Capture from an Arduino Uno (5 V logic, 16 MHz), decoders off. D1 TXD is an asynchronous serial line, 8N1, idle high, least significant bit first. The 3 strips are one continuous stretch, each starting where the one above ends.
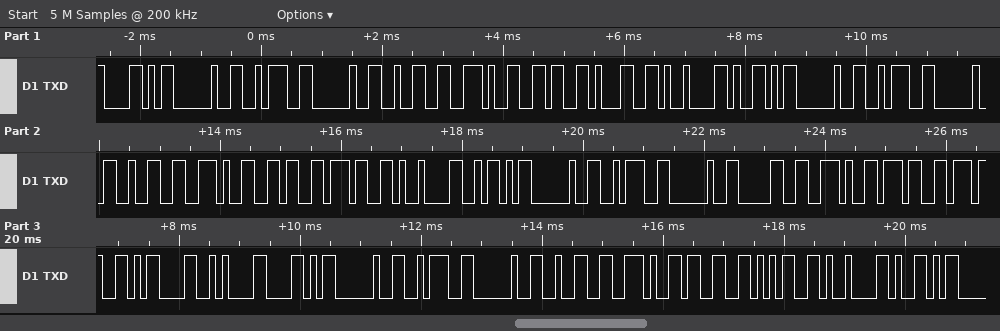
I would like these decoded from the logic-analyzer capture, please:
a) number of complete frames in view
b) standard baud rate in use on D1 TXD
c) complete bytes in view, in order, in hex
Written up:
38
9600 baud
58 20 3A 20 32 2E 36 31 09 59 20 3A 20 32 2E 36 37 09 5A 20 3A 20 30 2E 37 37 0D 0A 58 20 3A 20 32 2E 33 35 09 59
